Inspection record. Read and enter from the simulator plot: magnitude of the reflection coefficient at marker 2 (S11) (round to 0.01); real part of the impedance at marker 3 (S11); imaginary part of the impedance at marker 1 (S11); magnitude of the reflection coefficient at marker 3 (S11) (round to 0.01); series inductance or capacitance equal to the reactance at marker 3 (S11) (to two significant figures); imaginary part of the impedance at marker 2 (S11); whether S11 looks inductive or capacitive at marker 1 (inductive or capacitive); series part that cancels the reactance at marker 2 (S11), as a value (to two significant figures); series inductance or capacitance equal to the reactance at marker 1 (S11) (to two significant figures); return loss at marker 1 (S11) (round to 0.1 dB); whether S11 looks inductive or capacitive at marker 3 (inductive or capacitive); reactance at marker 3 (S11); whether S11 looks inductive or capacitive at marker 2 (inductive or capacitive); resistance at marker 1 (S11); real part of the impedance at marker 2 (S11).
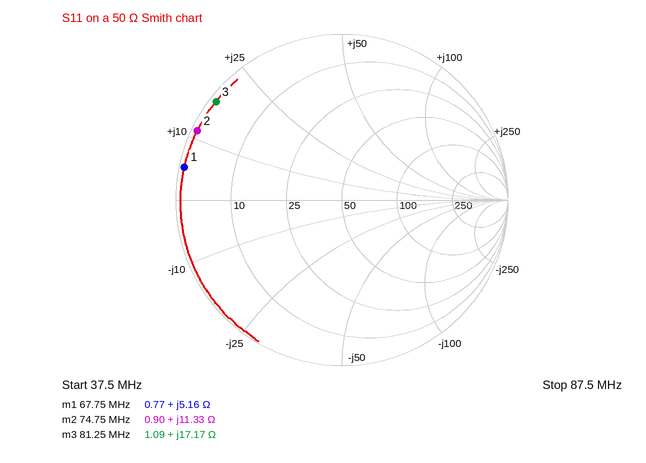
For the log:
0.97
1.09 Ω
+5.16 Ω
0.96
34 nH
+11.33 Ω
inductive
190 pF
12 nH
0.3 dB
inductive
+17.17 Ω
inductive
0.77 Ω
0.90 Ω
